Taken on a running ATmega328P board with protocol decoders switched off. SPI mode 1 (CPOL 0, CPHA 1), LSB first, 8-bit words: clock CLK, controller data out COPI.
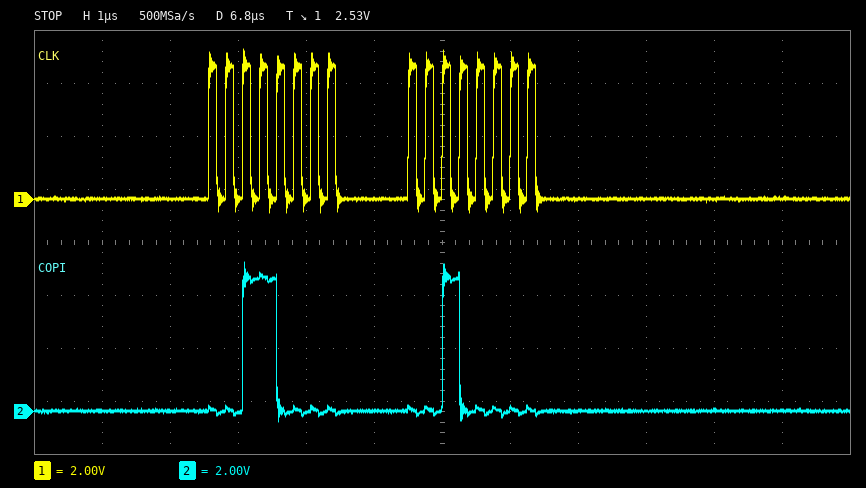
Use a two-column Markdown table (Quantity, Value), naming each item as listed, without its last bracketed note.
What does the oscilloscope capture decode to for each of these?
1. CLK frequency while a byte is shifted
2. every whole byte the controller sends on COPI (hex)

| Quantity | Value |
|---|---|
| CLK frequency while a byte is shifted | 4 MHz |
| every whole byte the controller sends on COPI | 0C 04 |
